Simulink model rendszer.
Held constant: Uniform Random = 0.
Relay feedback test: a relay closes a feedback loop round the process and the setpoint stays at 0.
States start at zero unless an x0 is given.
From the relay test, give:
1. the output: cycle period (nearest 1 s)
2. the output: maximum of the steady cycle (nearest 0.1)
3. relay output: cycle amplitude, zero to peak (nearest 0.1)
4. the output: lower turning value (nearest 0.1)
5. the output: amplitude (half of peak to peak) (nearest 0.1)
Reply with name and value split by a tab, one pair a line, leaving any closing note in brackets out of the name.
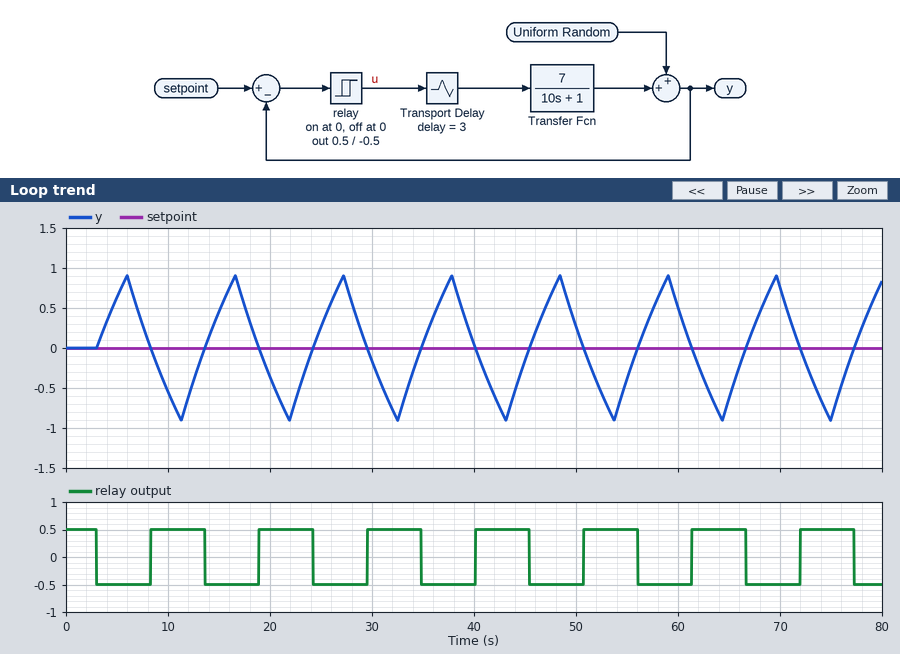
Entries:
the output: cycle period	11 s
the output: maximum of the steady cycle	0.9
relay output: cycle amplitude, zero to peak	0.5
the output: lower turning value	-0.9
the output: amplitude (half of peak to peak)	0.9
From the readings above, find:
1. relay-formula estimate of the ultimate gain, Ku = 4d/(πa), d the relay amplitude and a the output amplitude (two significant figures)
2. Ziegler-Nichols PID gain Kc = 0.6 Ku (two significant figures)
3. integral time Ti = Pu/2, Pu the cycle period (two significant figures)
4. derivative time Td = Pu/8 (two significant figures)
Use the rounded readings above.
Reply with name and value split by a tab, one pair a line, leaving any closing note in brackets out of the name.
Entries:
relay-formula estimate of the ultimate gain, Ku = 4d/(πa), d the relay amplitude and a the output amplitude	0.71
Ziegler-Nichols PID gain Kc = 0.6 Ku	0.43
integral time Ti = Pu/2, Pu the cycle period	5.5 s
derivative time Td = Pu/8	1.4 s
